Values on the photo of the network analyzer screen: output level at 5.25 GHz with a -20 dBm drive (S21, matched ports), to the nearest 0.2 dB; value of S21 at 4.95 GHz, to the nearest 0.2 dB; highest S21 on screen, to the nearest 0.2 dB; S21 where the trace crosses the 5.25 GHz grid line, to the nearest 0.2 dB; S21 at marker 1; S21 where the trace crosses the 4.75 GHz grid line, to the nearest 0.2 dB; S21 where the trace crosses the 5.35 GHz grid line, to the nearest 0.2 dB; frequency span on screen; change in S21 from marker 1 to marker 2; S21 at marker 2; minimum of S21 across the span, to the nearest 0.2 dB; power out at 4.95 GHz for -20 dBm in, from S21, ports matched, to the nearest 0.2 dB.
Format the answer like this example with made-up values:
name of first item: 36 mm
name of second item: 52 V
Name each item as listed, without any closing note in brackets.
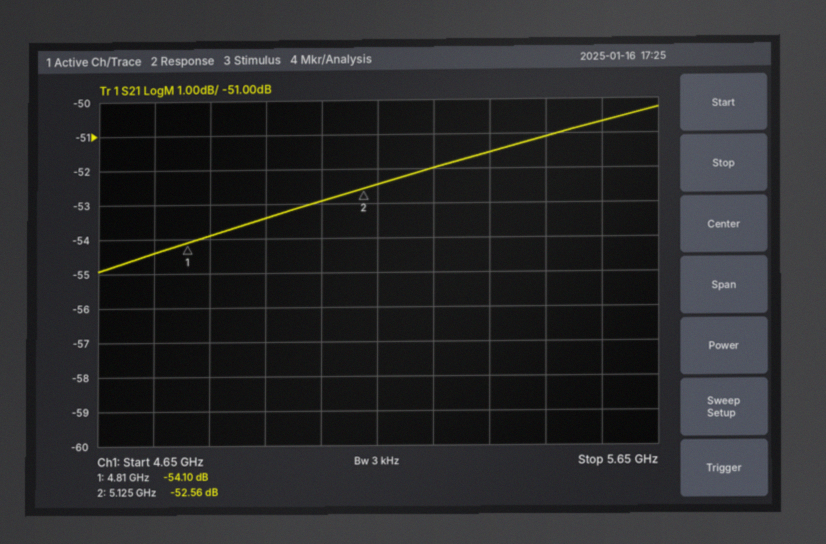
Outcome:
output level at 5.25 GHz with a -20 dBm drive (S21, matched ports), to the nearest 0.2 dB: -72.0 dBm
value of S21 at 4.95 GHz, to the nearest 0.2 dB: -53.4 dB
highest S21 on screen, to the nearest 0.2 dB: -50.2 dB
S21 where the trace crosses the 5.25 GHz grid line, to the nearest 0.2 dB: -52.0 dB
S21 at marker 1: -54.10 dB
S21 where the trace crosses the 4.75 GHz grid line, to the nearest 0.2 dB: -54.4 dB
S21 where the trace crosses the 5.35 GHz grid line, to the nearest 0.2 dB: -51.6 dB
frequency span on screen: 1 GHz
change in S21 from marker 1 to marker 2: 1.54 dB
S21 at marker 2: -52.56 dB
minimum of S21 across the span, to the nearest 0.2 dB: -55.0 dB
power out at 4.95 GHz for -20 dBm in, from S21, ports matched, to the nearest 0.2 dB: -73.4 dBm
